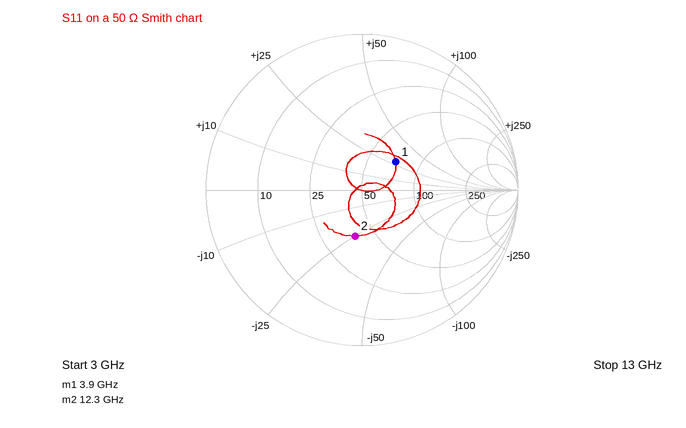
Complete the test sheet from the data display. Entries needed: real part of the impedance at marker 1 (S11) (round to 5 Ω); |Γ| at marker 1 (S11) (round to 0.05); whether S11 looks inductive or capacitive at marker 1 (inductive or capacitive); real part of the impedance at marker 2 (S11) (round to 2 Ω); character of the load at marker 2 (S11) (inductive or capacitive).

70 Ω
0.30
inductive
38 Ω
capacitive
